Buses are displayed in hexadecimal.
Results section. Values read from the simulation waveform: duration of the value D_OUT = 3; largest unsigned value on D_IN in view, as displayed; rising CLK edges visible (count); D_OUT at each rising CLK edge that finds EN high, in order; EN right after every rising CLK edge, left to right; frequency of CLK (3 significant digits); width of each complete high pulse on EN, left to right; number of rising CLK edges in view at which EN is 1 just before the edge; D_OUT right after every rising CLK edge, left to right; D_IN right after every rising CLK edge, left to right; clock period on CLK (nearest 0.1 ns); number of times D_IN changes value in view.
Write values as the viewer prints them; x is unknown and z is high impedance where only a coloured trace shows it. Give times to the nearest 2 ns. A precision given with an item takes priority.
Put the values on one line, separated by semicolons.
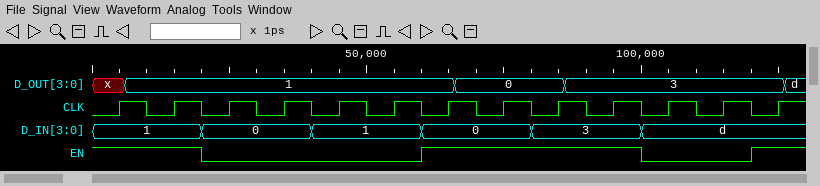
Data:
40 ns; d; 13; x, 1, 1, 0, 0, 3, 3; 1 1 0 0 0 0 1 1 1 1 0 0 1; 100 MHz; 40 ns; 7; x, 1, 1, 1, 1, 1, 1, 0, 0, 3, 3, 3, 3; 1, 1, 0, 0, 1, 1, 0, 0, 3, 3, d, d, d; 10 ns; 5
